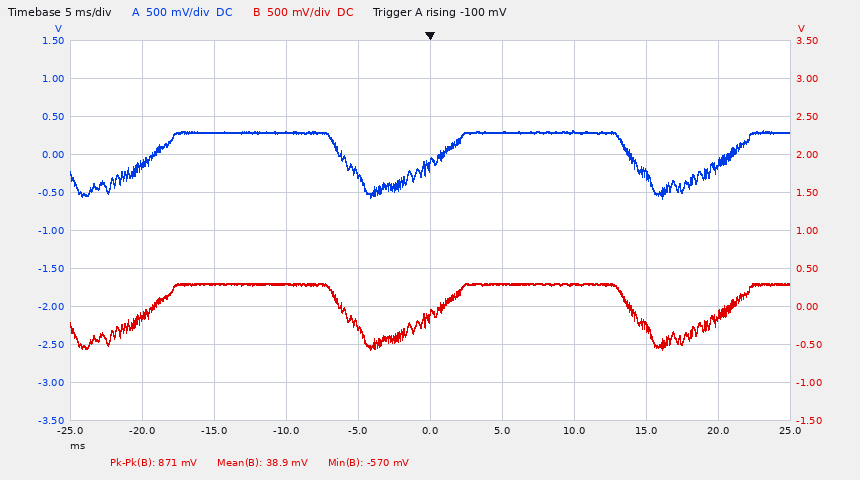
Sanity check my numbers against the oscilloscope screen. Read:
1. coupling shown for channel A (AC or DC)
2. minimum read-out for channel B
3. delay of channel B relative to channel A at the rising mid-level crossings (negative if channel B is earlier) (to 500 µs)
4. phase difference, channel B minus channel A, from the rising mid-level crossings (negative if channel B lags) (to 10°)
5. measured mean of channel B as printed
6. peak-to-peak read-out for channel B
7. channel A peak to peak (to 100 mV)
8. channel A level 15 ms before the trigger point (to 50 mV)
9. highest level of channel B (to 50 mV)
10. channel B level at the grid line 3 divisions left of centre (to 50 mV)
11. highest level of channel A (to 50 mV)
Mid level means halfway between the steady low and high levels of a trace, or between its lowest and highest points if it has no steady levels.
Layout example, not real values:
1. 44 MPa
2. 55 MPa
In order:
1. DC
2. -570 mV
3. 0.0 ms
4. 0°
5. 38.9 mV
6. 871 mV
7. 900 mV
8. 300 mV
9. 300 mV
10. 300 mV
11. 300 mV
